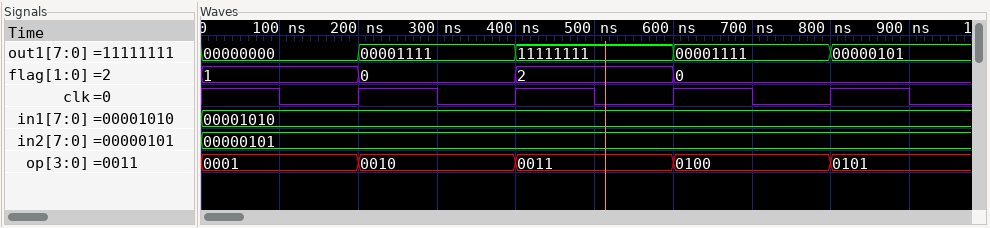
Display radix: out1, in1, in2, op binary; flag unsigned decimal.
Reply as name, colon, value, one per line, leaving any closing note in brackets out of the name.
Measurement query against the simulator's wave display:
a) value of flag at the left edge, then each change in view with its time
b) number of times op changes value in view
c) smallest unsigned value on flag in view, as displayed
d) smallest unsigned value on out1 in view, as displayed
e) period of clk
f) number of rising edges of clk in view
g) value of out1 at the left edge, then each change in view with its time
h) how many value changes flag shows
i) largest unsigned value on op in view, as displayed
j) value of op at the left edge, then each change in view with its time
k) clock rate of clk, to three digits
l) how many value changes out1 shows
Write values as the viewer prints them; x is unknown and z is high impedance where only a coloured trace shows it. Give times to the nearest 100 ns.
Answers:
value of flag at the left edge, then each change in view with its time: 1, 0 at 200 ns, 2 at 400 ns, 0 at 600 ns
number of times op changes value in view: 4
smallest unsigned value on flag in view, as displayed: 0
smallest unsigned value on out1 in view, as displayed: 00000000
period of clk: 200 ns
number of rising edges of clk in view: 4
value of out1 at the left edge, then each change in view with its time: 00000000, 00001111 at 200 ns, 11111111 at 400 ns, 00001111 at 600 ns, 00000101 at 800 ns
how many value changes flag shows: 3
largest unsigned value on op in view, as displayed: 0101
value of op at the left edge, then each change in view with its time: 0001, 0010 at 200 ns, 0011 at 400 ns, 0100 at 600 ns, 0101 at 800 ns
clock rate of clk, to three digits: 5.00 MHz
how many value changes out1 shows: 4
